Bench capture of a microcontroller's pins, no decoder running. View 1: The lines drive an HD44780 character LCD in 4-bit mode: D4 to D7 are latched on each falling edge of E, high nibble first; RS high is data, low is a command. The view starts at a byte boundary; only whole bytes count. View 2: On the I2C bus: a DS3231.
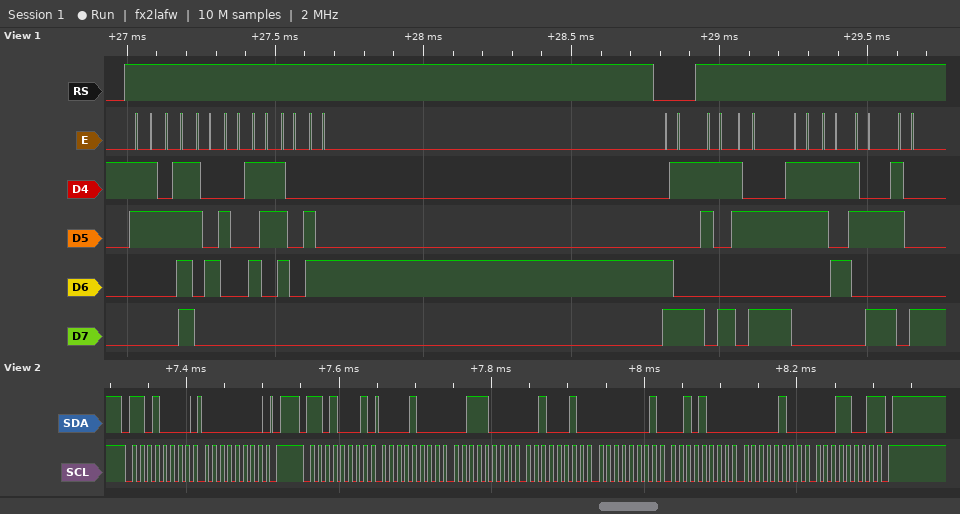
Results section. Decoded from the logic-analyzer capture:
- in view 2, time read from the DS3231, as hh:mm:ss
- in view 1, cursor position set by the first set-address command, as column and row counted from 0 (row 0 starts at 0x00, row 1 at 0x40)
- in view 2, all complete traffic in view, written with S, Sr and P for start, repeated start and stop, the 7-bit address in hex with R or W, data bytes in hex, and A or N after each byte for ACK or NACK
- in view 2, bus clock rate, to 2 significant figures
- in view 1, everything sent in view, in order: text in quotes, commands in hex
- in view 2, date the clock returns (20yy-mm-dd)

22:38:08
column 9, row 1
S 68W A 00 A P S 68R A 08 A 38 A 22 A 01 A 28 A 04 A 19 N P
100 kHz
"3/4 Spd" 0xC9 "9:35:8"
2019-04-28
